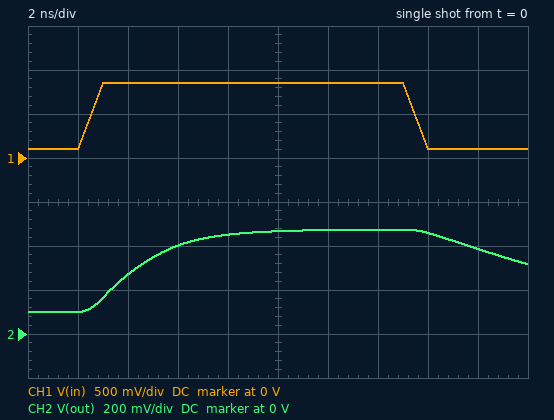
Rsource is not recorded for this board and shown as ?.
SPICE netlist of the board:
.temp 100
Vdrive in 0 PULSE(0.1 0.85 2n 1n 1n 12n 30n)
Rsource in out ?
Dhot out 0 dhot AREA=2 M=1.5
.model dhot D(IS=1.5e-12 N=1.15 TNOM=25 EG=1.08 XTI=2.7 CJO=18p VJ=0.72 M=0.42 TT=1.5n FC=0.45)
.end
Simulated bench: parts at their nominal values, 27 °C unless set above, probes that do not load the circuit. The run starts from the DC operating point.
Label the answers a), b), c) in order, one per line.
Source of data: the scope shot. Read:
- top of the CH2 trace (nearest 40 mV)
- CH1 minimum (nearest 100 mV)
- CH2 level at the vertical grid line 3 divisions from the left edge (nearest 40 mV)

a) 480 mV
b) 100 mV
c) 400 mV
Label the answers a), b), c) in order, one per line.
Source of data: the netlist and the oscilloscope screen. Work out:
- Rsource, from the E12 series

a) 82 Ω
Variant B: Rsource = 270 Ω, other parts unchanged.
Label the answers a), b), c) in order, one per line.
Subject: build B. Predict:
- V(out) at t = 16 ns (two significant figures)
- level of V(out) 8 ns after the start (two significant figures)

a) 400 mV
b) 290 mV
